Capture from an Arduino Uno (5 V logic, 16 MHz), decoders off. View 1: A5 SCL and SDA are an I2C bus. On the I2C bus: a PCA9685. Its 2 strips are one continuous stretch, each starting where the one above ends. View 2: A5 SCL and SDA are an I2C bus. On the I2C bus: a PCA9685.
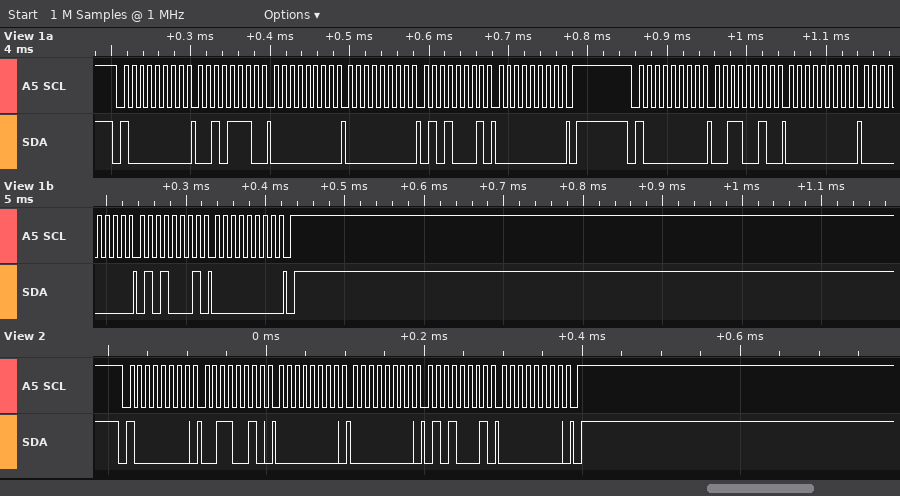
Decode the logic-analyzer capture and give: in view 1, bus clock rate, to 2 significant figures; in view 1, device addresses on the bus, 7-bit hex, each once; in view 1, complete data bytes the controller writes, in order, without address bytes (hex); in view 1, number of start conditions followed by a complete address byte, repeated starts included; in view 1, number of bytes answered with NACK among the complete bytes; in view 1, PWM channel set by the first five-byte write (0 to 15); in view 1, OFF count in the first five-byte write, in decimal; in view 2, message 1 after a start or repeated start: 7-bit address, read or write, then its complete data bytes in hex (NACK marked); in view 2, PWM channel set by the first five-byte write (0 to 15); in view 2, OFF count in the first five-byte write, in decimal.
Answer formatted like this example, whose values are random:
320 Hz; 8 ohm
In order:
100 kHz; 0x40; 2E 00 00 51 00 32 00 00 51 00; 2; 0; 10; 81; 0x40 write: 32 00 00 51 00; 11; 81
